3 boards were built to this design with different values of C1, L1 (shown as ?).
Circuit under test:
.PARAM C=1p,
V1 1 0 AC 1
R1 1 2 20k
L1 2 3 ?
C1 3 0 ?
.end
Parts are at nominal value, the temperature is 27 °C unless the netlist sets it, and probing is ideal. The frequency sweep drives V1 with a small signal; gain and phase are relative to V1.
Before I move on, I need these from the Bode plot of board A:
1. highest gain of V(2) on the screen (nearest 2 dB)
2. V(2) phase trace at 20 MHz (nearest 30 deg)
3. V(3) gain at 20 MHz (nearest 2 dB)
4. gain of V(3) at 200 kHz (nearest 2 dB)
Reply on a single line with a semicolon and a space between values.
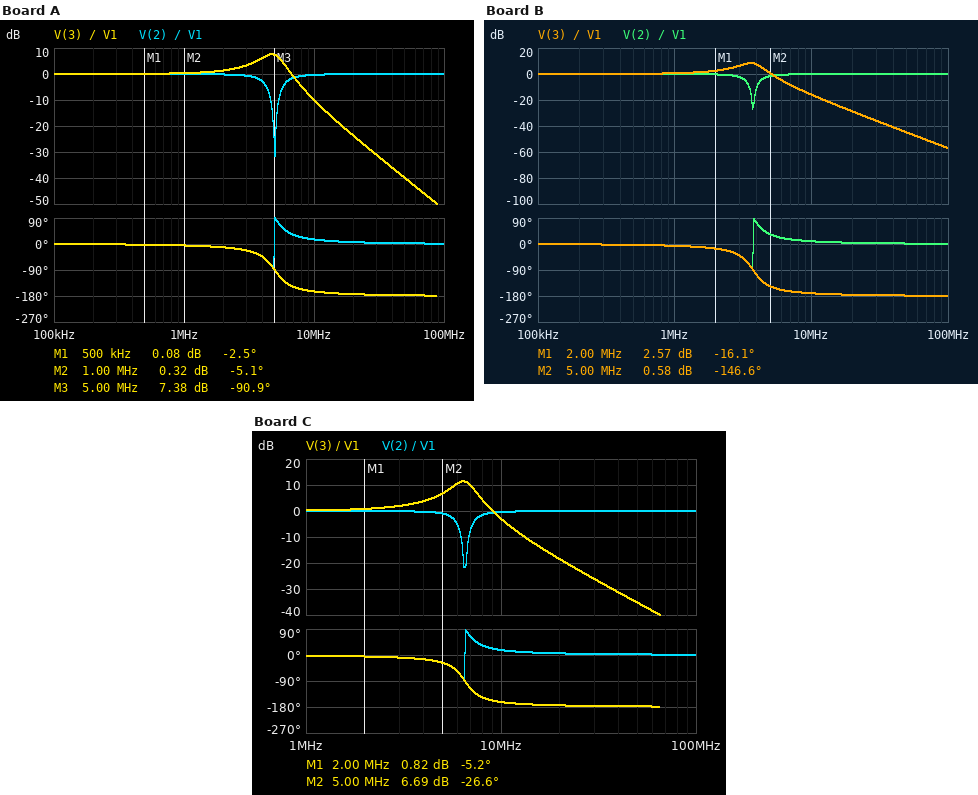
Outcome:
0 dB; 0 deg; -24 dB; 0 dB
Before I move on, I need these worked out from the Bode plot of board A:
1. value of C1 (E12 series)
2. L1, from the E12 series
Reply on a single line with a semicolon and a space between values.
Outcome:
680 fF; 1.5 mH
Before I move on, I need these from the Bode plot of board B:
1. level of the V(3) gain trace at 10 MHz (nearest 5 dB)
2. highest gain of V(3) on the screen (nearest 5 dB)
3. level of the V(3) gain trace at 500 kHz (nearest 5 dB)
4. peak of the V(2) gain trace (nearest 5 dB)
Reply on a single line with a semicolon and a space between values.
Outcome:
-15 dB; 10 dB; 0 dB; 0 dB
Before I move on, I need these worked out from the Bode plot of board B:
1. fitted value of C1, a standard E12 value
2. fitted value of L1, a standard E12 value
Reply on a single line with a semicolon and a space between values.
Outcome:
820 fF; 2.2 mH
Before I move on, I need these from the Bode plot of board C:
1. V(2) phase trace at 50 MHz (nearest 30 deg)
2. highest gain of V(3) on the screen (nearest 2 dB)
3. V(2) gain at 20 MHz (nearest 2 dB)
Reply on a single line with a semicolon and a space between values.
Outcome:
0 deg; 12 dB; 0 dB
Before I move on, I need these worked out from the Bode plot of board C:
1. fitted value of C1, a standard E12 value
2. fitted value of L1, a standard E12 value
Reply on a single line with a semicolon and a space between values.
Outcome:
330 fF; 1.8 mH
